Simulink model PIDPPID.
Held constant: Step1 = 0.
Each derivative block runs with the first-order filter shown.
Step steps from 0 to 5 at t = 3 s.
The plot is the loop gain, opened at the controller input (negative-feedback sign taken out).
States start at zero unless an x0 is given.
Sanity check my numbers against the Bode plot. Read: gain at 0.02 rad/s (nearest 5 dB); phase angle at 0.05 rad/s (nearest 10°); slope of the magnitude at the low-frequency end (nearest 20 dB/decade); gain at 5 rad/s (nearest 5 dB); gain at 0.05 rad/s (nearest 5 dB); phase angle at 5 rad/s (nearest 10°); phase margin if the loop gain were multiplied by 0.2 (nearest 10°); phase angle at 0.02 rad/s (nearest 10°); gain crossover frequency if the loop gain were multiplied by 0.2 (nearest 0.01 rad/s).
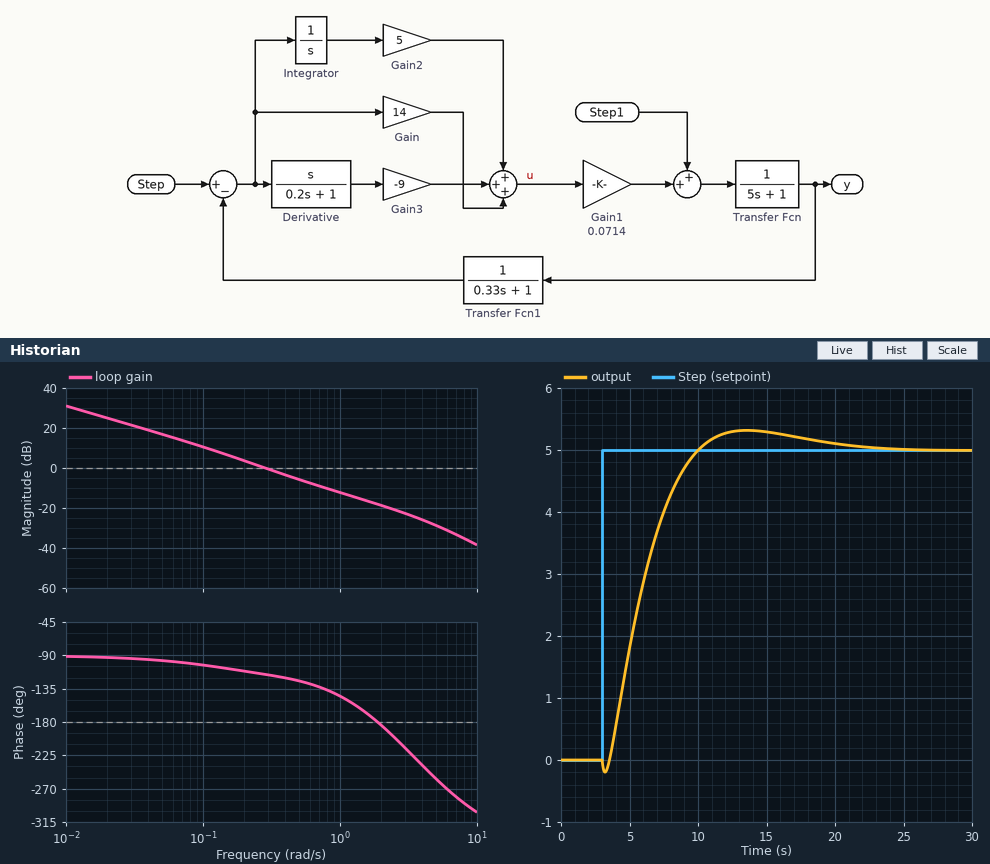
25 dB
-100°
-20 dB/decade
-30 dB
15 dB
-260°
80°
-90°
0.07 rad/s
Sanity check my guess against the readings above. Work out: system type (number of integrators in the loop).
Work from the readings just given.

1
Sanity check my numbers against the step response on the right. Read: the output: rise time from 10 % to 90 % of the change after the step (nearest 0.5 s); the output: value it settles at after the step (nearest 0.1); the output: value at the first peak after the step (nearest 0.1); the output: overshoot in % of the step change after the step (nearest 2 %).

4.5 s
5.0
5.3
6 %
